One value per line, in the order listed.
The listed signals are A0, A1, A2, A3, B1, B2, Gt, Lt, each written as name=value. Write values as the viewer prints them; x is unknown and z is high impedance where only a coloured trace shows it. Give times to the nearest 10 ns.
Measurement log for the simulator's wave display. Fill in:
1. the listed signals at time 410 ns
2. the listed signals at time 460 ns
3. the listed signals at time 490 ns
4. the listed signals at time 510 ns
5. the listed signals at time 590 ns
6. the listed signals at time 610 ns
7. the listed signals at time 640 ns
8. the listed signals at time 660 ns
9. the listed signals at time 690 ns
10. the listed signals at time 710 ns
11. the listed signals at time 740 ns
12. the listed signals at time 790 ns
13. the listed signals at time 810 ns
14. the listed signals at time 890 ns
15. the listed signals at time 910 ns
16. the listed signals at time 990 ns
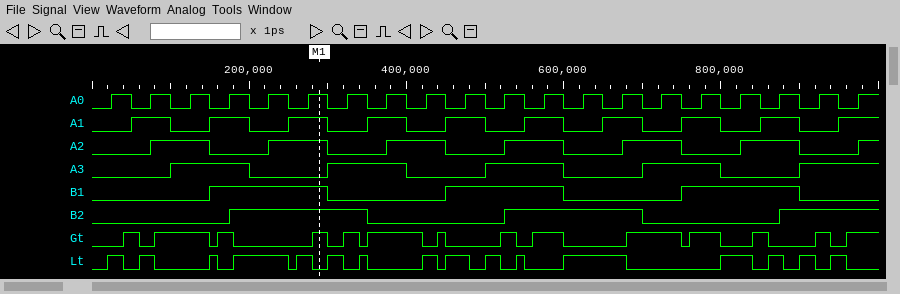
A0=0, A1=0, A2=1, A3=0, B1=0, B2=0, Gt=1, Lt=0
A0=0, A1=1, A2=0, A3=0, B1=1, B2=0, Gt=0, Lt=1
A0=1, A1=1, A2=0, A3=0, B1=1, B2=0, Gt=0, Lt=0
A0=0, A1=0, A2=0, A3=1, B1=1, B2=0, Gt=0, Lt=1
A0=1, A1=1, A2=1, A3=1, B1=1, B2=1, Gt=1, Lt=0
A0=0, A1=0, A2=0, A3=0, B1=0, B2=1, Gt=0, Lt=1
A0=1, A1=0, A2=0, A3=0, B1=0, B2=1, Gt=0, Lt=1
A0=0, A1=1, A2=0, A3=0, B1=0, B2=1, Gt=0, Lt=1
A0=1, A1=1, A2=1, A3=0, B1=0, B2=1, Gt=1, Lt=0
A0=0, A1=0, A2=1, A3=1, B1=0, B2=0, Gt=1, Lt=0
A0=1, A1=0, A2=1, A3=1, B1=0, B2=0, Gt=1, Lt=0
A0=1, A1=1, A2=0, A3=1, B1=1, B2=0, Gt=1, Lt=0
A0=0, A1=0, A2=0, A3=0, B1=1, B2=0, Gt=0, Lt=1
A0=1, A1=1, A2=1, A3=0, B1=1, B2=1, Gt=0, Lt=0
A0=0, A1=0, A2=0, A3=1, B1=0, B2=1, Gt=0, Lt=1
A0=1, A1=1, A2=1, A3=1, B1=0, B2=1, Gt=1, Lt=0
